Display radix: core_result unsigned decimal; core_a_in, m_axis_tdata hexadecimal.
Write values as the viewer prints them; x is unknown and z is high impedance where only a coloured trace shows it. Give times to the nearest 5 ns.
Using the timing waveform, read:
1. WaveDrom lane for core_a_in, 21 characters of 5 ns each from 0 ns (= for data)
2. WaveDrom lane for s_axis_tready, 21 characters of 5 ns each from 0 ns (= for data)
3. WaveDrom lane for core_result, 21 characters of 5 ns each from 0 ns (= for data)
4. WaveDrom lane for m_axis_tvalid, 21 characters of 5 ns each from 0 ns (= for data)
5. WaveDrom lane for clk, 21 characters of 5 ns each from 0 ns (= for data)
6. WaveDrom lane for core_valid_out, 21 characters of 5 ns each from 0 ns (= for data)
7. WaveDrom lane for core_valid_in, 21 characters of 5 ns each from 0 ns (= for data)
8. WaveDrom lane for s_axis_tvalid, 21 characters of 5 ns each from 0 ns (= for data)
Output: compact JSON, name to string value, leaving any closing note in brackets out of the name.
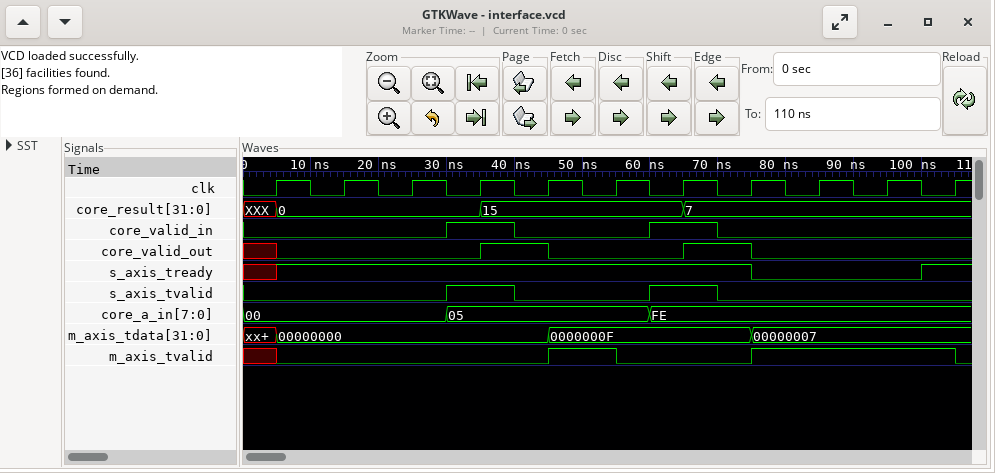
{"WaveDrom lane for core_a_in, 21 characters of 5 ns each from 0 ns": "{name: 'core_a_in', wave: '=.....=.....=........', data: '00 05 FE'}", "WaveDrom lane for s_axis_tready, 21 characters of 5 ns each from 0 ns": "{name: 's_axis_tready', wave: 'x1.............0....1'}", "WaveDrom lane for core_result, 21 characters of 5 ns each from 0 ns": "{name: 'core_result', wave: 'x=.....=.....=.......', data: '0 15 7'}", "WaveDrom lane for m_axis_tvalid, 21 characters of 5 ns each from 0 ns": "{name: 'm_axis_tvalid', wave: 'x0.......1.0...1.....'}", "WaveDrom lane for clk, 21 characters of 5 ns each from 0 ns": "{name: 'clk', wave: '010101010101010101010'}", "WaveDrom lane for core_valid_out, 21 characters of 5 ns each from 0 ns": "{name: 'core_valid_out', wave: 'x0.....1.0...1.0.....'}", "WaveDrom lane for core_valid_in, 21 characters of 5 ns each from 0 ns": "{name: 'core_valid_in', wave: '0.....1.0...1.0......'}", "WaveDrom lane for s_axis_tvalid, 21 characters of 5 ns each from 0 ns": "{name: 's_axis_tvalid', wave: '0.....1.0...1.0......'}"}
